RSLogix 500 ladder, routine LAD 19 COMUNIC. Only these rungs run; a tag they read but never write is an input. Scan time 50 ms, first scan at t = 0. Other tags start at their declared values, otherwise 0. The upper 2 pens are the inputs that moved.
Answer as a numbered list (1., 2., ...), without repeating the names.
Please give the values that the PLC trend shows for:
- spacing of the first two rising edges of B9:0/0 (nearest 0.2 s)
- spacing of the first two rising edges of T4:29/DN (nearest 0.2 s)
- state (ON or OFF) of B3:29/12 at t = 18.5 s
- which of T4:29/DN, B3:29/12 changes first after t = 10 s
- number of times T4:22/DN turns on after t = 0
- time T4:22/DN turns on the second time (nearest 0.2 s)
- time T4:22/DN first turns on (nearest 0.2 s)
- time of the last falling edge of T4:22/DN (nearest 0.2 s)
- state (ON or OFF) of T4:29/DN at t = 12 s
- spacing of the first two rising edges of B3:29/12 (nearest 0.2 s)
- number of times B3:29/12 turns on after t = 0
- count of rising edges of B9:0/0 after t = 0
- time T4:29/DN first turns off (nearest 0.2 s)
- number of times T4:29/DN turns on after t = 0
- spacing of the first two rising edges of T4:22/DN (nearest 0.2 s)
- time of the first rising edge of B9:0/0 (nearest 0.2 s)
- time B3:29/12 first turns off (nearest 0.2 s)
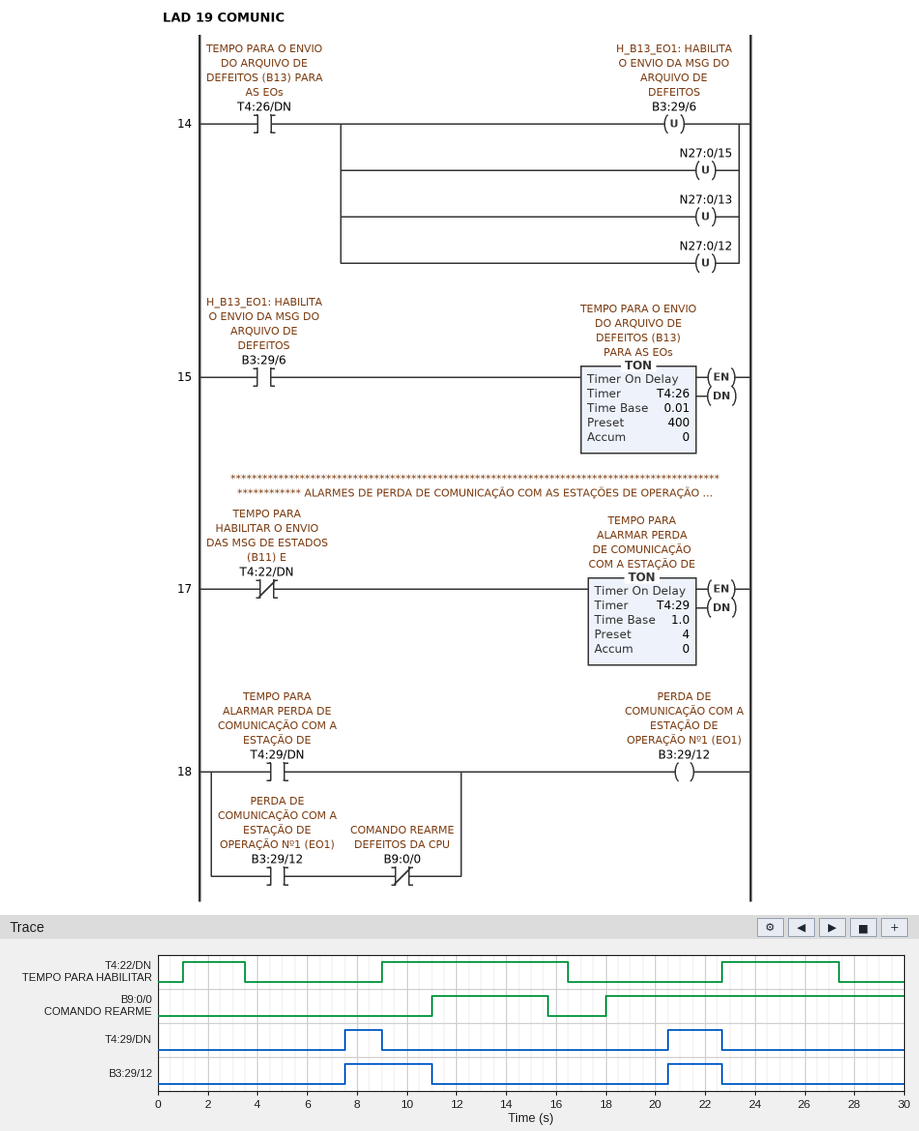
1. 7.0 s
2. 13.0 s
3. OFF
4. B3:29/12
5. 3
6. 9.0 s
7. 1.0 s
8. 27.4 s
9. OFF
10. 13.0 s
11. 2
12. 2
13. 9.0 s
14. 2
15. 8.0 s
16. 11.0 s
17. 11.0 s
